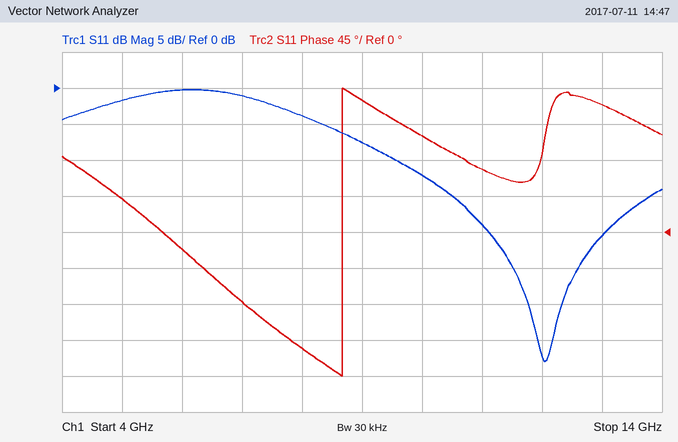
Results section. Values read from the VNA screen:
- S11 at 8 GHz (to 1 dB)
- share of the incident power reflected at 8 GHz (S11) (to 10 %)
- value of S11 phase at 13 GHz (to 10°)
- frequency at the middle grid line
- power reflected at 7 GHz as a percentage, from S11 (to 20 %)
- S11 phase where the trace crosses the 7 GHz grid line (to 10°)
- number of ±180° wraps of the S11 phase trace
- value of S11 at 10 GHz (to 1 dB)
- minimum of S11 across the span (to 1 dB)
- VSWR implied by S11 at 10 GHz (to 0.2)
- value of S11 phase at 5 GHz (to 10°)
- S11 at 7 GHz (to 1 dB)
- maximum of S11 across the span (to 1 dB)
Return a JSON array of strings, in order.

["-4 dB", "40 %", "160°", "9 GHz", "80 %", "-90°", "1", "-12 dB", "-38 dB", "1.6", "40°", "-1 dB", "0 dB"]
